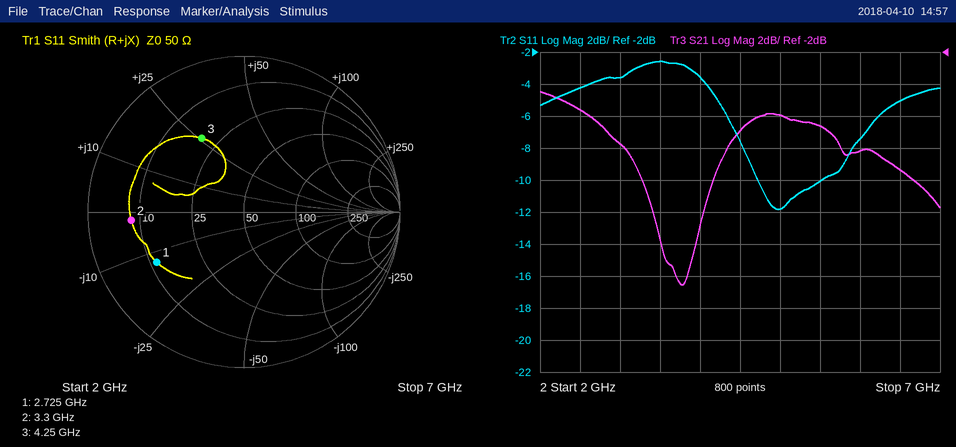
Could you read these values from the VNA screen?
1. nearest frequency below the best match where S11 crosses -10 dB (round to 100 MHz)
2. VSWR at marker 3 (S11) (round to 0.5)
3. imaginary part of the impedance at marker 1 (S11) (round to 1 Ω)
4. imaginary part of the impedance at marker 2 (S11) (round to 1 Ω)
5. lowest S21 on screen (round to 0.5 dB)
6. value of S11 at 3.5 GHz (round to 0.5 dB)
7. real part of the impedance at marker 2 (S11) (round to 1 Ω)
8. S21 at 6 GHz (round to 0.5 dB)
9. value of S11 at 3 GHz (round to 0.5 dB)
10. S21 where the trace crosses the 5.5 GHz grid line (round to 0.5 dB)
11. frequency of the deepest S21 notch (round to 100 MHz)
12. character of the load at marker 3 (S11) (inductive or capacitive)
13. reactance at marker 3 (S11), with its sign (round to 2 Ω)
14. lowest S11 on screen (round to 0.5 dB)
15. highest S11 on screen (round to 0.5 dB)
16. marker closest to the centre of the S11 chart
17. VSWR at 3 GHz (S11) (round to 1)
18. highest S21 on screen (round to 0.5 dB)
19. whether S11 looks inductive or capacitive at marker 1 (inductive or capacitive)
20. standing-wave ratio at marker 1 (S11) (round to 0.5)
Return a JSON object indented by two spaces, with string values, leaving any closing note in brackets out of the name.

{
  "nearest frequency below the best match where S11 crosses -10 dB": "4.7 GHz",
  "VSWR at marker 3 (S11)": "3.5",
  "imaginary part of the impedance at marker 1 (S11)": "-13 Ω",
  "imaginary part of the impedance at marker 2 (S11)": "-2 Ω",
  "lowest S21 on screen": "-16.5 dB",
  "value of S11 at 3.5 GHz": "-2.5 dB",
  "real part of the impedance at marker 2 (S11)": "8 Ω",
  "S21 at 6 GHz": "-8.0 dB",
  "value of S11 at 3 GHz": "-3.5 dB",
  "S21 where the trace crosses the 5.5 GHz grid line": "-6.5 dB",
  "frequency of the deepest S21 notch": "3.8 GHz",
  "character of the load at marker 3 (S11)": "inductive",
  "reactance at marker 3 (S11), with its sign": "+26 Ω",
  "lowest S11 on screen": "-12.0 dB",
  "highest S11 on screen": "-2.5 dB",
  "marker closest to the centre of the S11 chart": "marker 3",
  "VSWR at 3 GHz (S11)": "5",
  "highest S21 on screen": "-4.5 dB",
  "whether S11 looks inductive or capacitive at marker 1": "capacitive",
  "standing-wave ratio at marker 1 (S11)": "4.5"
}
